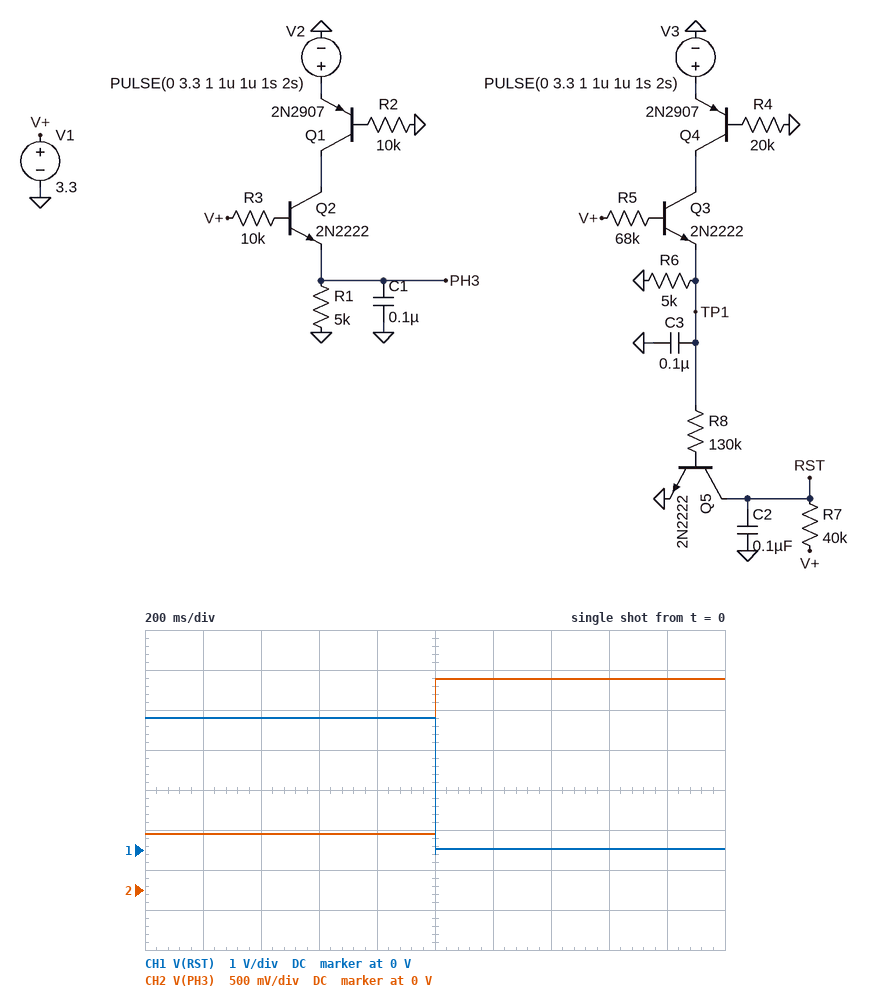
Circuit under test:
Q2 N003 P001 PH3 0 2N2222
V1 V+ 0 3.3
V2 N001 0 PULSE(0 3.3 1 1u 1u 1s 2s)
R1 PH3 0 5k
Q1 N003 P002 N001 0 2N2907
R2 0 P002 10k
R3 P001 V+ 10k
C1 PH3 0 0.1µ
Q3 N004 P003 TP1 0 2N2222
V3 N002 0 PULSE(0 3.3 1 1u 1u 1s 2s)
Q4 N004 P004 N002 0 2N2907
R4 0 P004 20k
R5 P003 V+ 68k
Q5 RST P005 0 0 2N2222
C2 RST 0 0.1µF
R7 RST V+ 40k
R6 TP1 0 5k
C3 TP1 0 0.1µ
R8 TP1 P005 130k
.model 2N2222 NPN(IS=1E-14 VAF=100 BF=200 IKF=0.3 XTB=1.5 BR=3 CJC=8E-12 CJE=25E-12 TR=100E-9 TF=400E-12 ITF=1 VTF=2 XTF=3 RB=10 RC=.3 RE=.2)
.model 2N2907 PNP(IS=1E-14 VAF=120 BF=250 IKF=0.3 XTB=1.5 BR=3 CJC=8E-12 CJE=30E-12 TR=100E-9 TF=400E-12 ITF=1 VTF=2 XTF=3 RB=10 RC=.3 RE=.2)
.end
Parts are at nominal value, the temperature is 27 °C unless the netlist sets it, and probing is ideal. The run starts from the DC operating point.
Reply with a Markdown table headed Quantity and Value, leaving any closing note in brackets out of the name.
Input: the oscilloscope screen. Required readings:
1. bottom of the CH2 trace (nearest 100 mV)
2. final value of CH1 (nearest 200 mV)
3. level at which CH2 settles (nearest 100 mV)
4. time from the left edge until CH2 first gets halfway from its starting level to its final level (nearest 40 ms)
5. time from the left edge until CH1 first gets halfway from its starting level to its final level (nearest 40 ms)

| Quantity | Value |
|---|---|
| bottom of the CH2 trace | 700 mV |
| final value of CH1 | 0 V |
| level at which CH2 settles | 2.6 V |
| time from the left edge until CH2 first gets halfway from its starting level to its final level | 1.00 s |
| time from the left edge until CH1 first gets halfway from its starting level to its final level | 1.00 s |
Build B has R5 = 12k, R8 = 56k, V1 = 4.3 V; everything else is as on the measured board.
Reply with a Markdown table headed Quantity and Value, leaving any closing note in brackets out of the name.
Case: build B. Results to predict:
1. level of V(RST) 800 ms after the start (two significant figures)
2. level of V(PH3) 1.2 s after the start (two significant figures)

| Quantity | Value |
|---|---|
| level of V(RST) 800 ms after the start | 61 mV |
| level of V(PH3) 1.2 s after the start | 3.2 V |
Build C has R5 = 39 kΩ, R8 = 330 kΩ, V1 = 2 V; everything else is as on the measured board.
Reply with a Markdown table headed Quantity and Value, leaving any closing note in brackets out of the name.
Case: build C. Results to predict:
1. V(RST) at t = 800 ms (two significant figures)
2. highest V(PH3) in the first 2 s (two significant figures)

| Quantity | Value |
|---|---|
| V(RST) at t = 800 ms | 2.0 V |
| highest V(PH3) in the first 2 s | 1.4 V |
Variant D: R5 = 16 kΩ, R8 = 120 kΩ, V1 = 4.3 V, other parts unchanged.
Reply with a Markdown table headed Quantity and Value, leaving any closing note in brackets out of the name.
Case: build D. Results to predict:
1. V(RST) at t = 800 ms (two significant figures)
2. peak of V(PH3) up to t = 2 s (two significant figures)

| Quantity | Value |
|---|---|
| V(RST) at t = 800 ms | 110 mV |
| peak of V(PH3) up to t = 2 s | 3.2 V |
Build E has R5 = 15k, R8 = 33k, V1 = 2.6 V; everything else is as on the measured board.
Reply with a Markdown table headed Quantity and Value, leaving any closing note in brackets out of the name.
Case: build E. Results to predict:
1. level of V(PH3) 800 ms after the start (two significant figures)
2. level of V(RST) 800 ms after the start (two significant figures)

| Quantity | Value |
|---|---|
| level of V(PH3) 800 ms after the start | 590 mV |
| level of V(RST) 800 ms after the start | 2.5 V |
